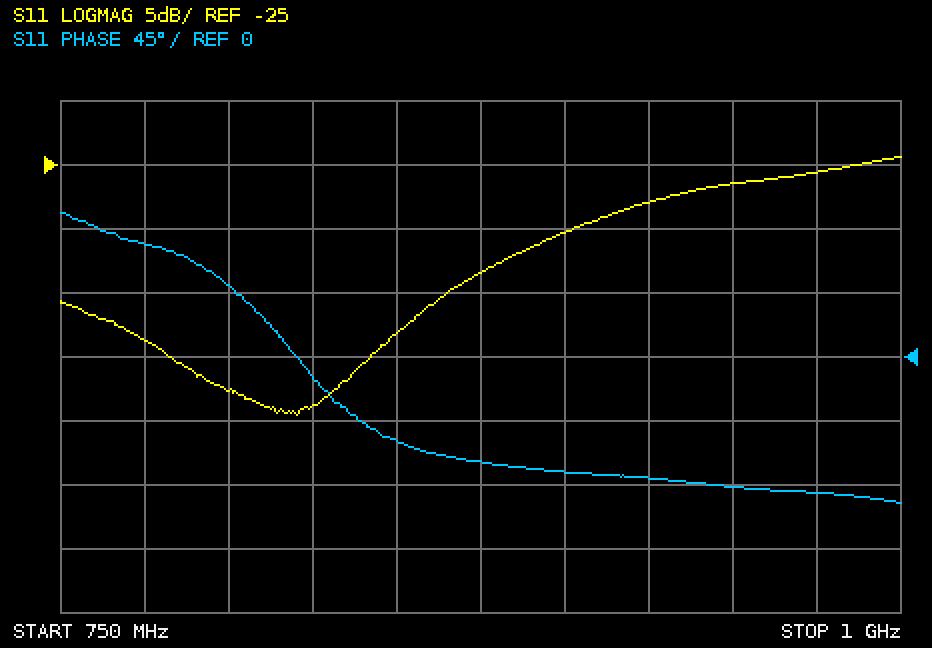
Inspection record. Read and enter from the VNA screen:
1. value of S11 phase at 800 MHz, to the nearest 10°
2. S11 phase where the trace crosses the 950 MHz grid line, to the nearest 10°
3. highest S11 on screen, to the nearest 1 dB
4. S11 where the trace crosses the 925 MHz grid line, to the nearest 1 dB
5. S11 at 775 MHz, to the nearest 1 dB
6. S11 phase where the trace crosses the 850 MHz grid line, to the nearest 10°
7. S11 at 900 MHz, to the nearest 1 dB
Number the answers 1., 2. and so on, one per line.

1. 50°
2. -90°
3. -24 dB
4. -28 dB
5. -39 dB
6. -60°
7. -30 dB
